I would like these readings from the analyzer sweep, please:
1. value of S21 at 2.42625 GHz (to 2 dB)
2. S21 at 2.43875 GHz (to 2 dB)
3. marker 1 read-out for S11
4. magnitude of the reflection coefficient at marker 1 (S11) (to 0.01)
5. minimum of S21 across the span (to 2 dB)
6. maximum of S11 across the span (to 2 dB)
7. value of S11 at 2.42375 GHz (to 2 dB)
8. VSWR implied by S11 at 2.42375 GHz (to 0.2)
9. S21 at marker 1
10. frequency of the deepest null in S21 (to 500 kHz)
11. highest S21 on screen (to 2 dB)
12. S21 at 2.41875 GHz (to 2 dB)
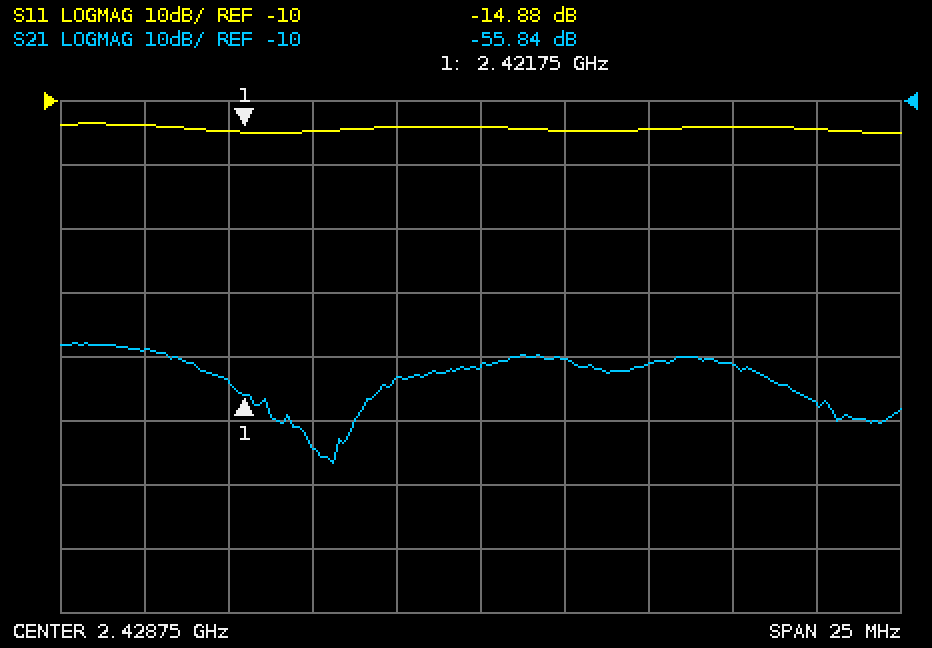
-54 dB
-58 dB
-14.88 dB
0.18
-66 dB
-14 dB
-14 dB
1.4
-55.84 dB
2.4245 GHz
-48 dB
-48 dB
